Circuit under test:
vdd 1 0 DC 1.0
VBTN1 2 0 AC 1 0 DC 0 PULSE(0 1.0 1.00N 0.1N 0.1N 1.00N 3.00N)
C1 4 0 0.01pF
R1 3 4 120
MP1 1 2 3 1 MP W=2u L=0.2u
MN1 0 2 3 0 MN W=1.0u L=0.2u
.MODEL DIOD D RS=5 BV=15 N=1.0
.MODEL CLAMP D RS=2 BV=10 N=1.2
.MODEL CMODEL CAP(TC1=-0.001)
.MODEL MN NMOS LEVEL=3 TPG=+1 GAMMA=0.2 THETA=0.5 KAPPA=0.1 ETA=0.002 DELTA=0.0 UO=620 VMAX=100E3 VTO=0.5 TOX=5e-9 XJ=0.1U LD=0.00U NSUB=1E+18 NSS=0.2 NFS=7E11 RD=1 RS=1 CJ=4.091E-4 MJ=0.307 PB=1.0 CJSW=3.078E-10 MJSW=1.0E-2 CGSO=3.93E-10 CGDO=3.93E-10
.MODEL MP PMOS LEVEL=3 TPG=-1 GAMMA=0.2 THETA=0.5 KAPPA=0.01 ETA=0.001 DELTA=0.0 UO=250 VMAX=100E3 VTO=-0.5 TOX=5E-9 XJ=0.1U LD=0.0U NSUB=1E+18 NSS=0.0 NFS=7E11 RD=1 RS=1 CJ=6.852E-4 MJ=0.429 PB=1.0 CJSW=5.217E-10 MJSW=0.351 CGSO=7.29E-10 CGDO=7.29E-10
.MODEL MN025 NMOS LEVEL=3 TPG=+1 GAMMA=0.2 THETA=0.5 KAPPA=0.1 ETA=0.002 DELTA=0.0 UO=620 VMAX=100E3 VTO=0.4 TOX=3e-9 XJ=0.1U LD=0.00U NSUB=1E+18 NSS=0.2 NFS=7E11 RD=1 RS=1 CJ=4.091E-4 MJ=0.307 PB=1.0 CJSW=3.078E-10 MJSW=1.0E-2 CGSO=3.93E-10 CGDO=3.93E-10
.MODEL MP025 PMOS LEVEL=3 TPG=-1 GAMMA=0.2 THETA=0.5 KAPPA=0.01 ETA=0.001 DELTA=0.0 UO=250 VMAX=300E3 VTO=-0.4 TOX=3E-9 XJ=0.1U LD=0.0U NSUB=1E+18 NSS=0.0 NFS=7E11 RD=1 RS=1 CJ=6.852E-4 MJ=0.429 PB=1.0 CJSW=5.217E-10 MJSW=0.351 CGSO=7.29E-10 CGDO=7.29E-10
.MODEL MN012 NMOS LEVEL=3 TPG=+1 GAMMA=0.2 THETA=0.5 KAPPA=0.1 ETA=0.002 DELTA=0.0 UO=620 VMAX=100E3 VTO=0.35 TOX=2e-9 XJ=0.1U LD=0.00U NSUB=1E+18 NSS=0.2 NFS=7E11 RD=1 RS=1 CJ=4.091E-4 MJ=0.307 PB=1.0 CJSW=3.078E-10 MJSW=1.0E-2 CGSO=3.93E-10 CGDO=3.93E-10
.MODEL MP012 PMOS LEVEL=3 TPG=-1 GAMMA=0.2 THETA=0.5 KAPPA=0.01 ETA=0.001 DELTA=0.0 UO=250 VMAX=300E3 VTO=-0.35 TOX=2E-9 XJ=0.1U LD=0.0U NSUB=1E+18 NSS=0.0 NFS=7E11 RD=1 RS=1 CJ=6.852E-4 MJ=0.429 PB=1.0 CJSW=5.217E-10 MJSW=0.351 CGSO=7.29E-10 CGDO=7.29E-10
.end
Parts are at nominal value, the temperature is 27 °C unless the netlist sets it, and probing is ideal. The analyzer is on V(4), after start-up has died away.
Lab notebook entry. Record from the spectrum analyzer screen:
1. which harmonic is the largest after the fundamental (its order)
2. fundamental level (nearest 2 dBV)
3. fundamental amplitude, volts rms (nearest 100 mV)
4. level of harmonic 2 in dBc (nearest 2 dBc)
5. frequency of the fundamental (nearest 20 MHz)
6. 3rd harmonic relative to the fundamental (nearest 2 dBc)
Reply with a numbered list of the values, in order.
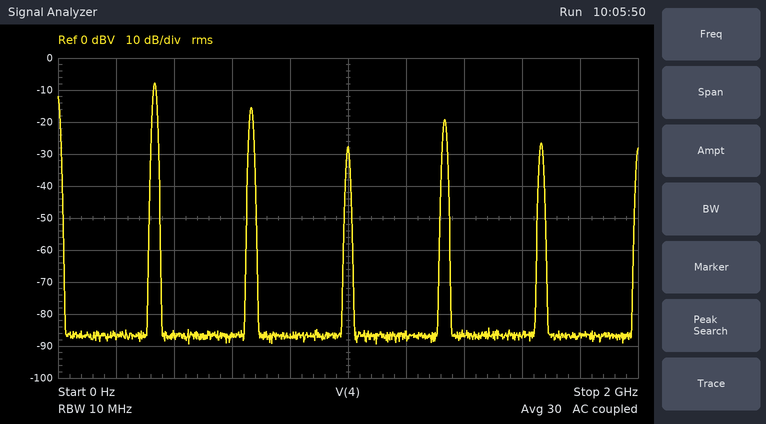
1. 2
2. -8 dBV
3. 400 mV
4. -8 dBc
5. 340 MHz
6. -20 dBc
